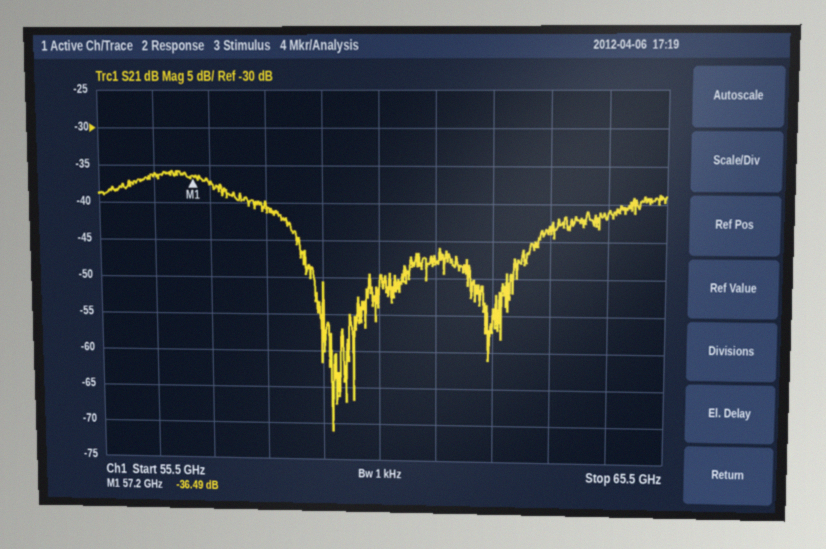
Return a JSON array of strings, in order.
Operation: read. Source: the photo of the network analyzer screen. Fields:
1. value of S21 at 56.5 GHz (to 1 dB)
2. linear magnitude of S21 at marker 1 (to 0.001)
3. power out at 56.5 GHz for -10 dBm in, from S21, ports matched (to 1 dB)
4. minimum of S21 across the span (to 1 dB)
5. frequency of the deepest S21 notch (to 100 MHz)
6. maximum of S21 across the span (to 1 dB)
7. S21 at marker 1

["-36 dB", "0.015", "-46 dBm", "-71 dB", "59.7 GHz", "-36 dB", "-36.49 dB"]
